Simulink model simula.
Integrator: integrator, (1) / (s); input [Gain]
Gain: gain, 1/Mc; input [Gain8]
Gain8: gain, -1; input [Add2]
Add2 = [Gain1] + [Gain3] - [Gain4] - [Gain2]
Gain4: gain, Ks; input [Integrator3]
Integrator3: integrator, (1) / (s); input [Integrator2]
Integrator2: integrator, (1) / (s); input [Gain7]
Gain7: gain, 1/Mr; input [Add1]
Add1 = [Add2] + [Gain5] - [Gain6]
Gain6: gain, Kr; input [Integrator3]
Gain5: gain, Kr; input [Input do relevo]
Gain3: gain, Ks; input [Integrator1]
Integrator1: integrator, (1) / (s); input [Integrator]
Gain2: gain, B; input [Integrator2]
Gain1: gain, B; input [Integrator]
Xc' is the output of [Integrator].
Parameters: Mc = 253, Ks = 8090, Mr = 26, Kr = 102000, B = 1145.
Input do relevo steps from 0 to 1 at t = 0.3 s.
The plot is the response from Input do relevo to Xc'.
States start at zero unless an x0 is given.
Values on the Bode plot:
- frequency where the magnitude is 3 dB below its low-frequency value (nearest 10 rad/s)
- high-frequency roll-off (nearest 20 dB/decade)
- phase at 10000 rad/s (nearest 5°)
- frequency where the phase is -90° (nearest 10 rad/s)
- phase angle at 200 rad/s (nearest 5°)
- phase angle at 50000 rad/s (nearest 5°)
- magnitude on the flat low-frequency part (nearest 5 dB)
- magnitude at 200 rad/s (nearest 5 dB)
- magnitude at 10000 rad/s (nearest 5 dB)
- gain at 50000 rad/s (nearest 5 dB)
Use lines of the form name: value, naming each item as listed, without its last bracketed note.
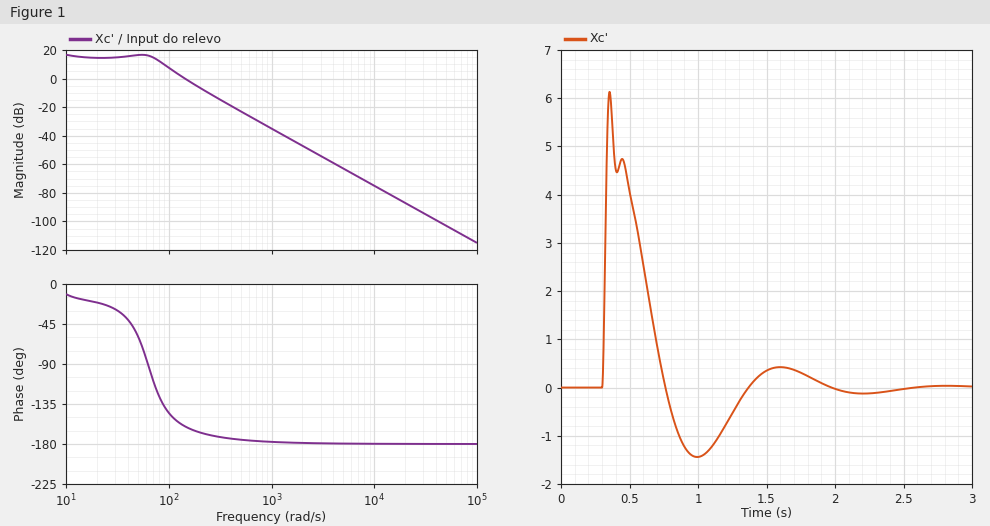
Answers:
frequency where the magnitude is 3 dB below its low-frequency value: 80 rad/s
high-frequency roll-off: -40 dB/decade
phase at 10000 rad/s: -180°
frequency where the phase is -90°: 60 rad/s
phase angle at 200 rad/s: -165°
phase angle at 50000 rad/s: -180°
magnitude on the flat low-frequency part: 15 dB
magnitude at 200 rad/s: -5 dB
magnitude at 10000 rad/s: -75 dB
gain at 50000 rad/s: -105 dB
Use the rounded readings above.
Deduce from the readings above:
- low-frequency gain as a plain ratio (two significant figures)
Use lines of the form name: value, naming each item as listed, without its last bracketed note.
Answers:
low-frequency gain as a plain ratio: 5.6
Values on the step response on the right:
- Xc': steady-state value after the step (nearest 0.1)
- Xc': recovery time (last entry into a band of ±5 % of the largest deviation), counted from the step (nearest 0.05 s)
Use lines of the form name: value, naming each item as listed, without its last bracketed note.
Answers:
Xc': steady-state value after the step: 0.0
Xc': recovery time (last entry into a band of ±5 % of the largest deviation), counted from the step: 1.45 s
